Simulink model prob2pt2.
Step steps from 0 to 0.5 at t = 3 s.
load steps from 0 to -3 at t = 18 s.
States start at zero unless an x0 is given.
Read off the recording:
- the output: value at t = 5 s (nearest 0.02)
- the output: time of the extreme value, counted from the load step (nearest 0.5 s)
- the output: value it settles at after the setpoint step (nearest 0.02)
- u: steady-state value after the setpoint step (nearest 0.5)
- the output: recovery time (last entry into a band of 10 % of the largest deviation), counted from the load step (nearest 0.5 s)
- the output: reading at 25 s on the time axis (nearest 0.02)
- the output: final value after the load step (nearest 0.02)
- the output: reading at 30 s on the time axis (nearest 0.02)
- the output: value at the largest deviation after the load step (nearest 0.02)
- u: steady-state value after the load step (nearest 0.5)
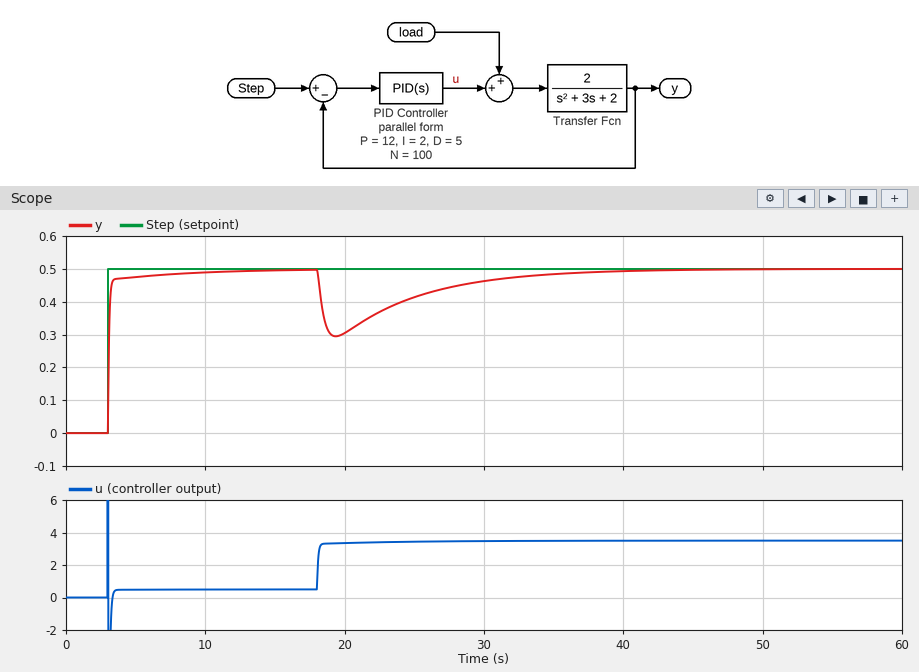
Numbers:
0.48
1.5 s
0.50
0.5
15.5 s
0.42
0.50
0.46
0.30
3.5
